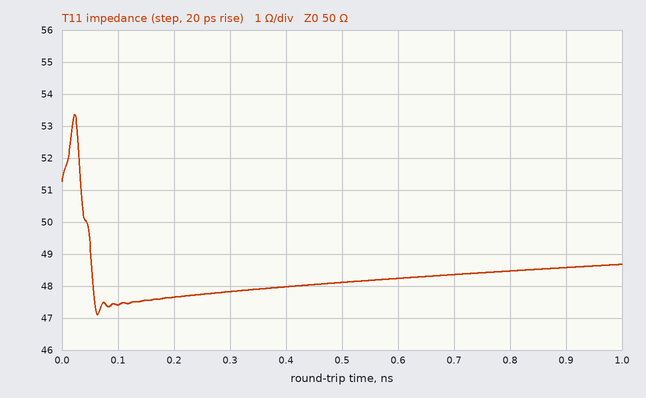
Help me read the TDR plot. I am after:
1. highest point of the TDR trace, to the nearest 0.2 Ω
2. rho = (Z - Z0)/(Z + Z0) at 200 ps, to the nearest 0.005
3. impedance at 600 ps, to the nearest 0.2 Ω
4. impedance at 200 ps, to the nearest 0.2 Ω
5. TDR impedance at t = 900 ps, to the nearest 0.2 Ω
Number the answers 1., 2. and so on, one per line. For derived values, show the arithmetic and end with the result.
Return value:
1. 53.4 Ω
2. (47.6 − 50)/(47.6 + 50) ≈ -0.025
3. 48.2 Ω
4. 47.6 Ω
5. 48.6 Ω
